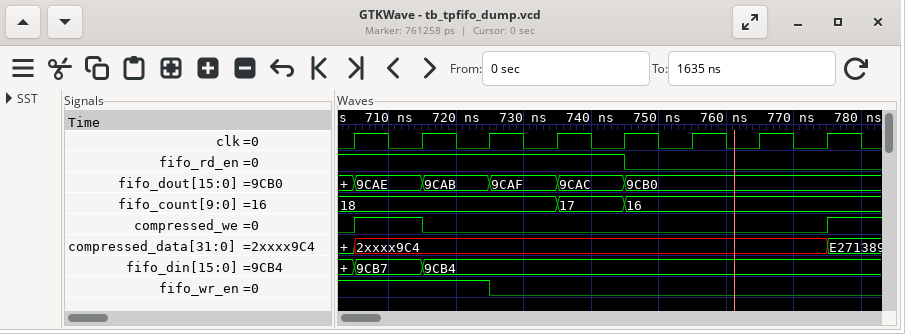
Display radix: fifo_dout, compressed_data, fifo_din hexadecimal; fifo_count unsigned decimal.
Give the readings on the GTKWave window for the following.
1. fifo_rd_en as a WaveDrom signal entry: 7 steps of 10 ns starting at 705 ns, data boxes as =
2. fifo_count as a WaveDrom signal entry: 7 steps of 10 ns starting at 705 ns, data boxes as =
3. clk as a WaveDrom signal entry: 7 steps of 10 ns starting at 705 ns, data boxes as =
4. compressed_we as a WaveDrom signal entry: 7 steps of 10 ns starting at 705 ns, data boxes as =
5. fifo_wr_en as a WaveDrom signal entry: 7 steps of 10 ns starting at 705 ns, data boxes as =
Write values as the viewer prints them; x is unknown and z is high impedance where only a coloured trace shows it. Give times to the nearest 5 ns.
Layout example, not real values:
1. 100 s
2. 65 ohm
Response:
1. {name: 'fifo_rd_en', wave: '1...0..'}
2. {name: 'fifo_count', wave: '=..==..', data: '18 17 16'}
3. {name: 'clk', wave: 'p......'}
4. {name: 'compressed_we', wave: '10.....'}
5. {name: 'fifo_wr_en', wave: '1.0....'}
